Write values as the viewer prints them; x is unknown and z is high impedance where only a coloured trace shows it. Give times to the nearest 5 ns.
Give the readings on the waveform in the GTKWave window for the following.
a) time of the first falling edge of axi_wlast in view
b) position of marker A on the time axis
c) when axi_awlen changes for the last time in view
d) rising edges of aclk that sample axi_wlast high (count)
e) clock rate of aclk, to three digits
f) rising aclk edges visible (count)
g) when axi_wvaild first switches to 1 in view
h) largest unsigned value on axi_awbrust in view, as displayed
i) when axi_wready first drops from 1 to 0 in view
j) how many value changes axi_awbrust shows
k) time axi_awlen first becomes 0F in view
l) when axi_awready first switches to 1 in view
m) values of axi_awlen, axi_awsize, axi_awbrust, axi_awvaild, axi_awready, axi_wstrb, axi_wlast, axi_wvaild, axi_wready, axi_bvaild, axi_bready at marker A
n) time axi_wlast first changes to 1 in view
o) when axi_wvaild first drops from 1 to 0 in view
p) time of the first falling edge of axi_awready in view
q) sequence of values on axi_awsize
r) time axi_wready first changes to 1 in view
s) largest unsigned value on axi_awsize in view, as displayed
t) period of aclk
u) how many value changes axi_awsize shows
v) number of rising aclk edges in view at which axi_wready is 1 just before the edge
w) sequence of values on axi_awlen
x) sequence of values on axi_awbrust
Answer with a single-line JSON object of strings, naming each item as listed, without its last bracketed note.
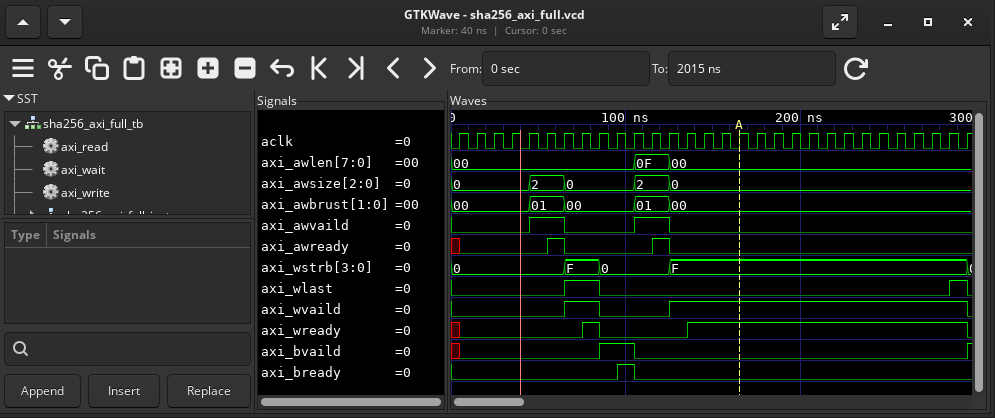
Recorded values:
{"time of the first falling edge of axi_wlast in view": "85 ns", "position of marker A on the time axis": "165 ns", "when axi_awlen changes for the last time in view": "125 ns", "rising edges of aclk that sample axi_wlast high": "3", "clock rate of aclk, to three digits": "100 MHz", "rising aclk edges visible": "30", "when axi_wvaild first switches to 1 in view": "65 ns", "largest unsigned value on axi_awbrust in view, as displayed": "01", "when axi_wready first drops from 1 to 0 in view": "85 ns", "how many value changes axi_awbrust shows": "4", "time axi_awlen first becomes 0F in view": "105 ns", "when axi_awready first switches to 1 in view": "55 ns", "values of axi_awlen, axi_awsize, axi_awbrust, axi_awvaild, axi_awready, axi_wstrb, axi_wlast, axi_wvaild, axi_wready, axi_bvaild, axi_bready at marker A": "axi_awlen=00, axi_awsize=0, axi_awbrust=00, axi_awvaild=0, axi_awready=0, axi_wstrb=F, axi_wlast=0, axi_wvaild=1, axi_wready=1, axi_bvaild=0, axi_bready=0", "time axi_wlast first changes to 1 in view": "65 ns", "when axi_wvaild first drops from 1 to 0 in view": "85 ns", "time of the first falling edge of axi_awready in view": "65 ns", "sequence of values on axi_awsize": "0, 2, 0, 2, 0", "time axi_wready first changes to 1 in view": "75 ns", "largest unsigned value on axi_awsize in view, as displayed": "2", "period of aclk": "10 ns", "how many value changes axi_awsize shows": "4", "number of rising aclk edges in view at which axi_wready is 1 just before the edge": "17", "sequence of values on axi_awlen": "00, 0F, 00", "sequence of values on axi_awbrust": "00, 01, 00, 01, 00"}
